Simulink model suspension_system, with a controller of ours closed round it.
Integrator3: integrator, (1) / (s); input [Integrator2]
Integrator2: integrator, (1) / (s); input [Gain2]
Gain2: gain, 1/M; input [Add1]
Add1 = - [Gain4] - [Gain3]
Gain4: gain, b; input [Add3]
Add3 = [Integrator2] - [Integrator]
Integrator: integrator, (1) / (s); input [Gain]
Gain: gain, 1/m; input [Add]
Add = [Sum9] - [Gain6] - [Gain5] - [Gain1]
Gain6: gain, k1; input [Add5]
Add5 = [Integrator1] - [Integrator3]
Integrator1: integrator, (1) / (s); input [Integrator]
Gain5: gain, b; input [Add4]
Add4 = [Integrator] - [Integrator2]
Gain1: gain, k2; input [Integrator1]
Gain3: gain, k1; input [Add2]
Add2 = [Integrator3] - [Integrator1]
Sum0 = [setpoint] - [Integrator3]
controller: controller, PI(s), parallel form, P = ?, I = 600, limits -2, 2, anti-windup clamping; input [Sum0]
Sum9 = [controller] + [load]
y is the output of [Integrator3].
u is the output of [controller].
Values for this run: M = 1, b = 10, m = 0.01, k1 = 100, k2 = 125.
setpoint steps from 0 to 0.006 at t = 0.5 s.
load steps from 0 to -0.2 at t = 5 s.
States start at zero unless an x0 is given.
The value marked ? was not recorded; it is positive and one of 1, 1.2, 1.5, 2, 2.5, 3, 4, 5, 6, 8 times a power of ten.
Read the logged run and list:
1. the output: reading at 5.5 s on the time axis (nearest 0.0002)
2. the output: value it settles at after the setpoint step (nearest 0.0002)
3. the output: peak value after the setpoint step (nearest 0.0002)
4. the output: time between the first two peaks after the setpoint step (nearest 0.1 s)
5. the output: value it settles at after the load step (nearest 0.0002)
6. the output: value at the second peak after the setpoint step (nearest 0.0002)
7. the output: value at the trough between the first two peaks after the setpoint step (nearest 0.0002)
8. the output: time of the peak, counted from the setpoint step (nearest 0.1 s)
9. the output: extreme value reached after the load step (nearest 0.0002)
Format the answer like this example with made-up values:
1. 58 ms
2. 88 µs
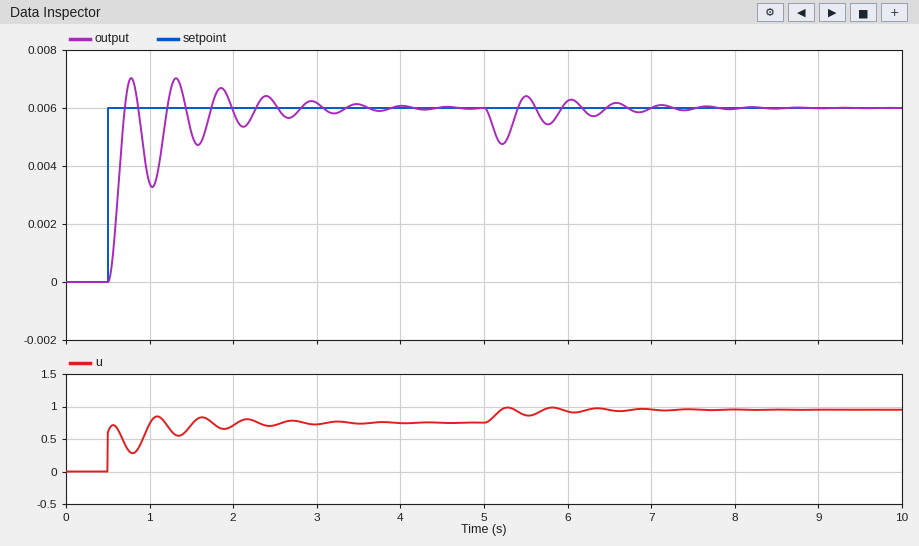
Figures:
1. 0.0064
2. 0.0060
3. 0.0070
4. 0.5 s
5. 0.0060
6. 0.0070
7. 0.0032
8. 0.3 s
9. 0.0048
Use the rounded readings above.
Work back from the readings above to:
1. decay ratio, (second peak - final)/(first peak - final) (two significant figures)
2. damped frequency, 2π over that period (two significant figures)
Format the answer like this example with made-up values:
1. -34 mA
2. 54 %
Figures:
1. 1.0
2. 13 rad/s
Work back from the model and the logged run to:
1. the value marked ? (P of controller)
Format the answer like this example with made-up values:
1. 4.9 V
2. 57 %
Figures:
1. 100
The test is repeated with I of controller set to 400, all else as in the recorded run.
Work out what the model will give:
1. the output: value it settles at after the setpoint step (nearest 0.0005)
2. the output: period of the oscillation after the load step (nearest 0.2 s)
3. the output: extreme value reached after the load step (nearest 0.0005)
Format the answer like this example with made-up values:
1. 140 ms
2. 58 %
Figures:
1. 0.0060
2. 0.6 s
3. 0.0045
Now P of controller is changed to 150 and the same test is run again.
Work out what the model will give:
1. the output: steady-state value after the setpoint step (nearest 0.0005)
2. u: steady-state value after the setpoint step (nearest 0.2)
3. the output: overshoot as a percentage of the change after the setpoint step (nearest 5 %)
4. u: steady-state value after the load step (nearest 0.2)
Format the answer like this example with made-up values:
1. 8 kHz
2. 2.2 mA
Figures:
1. 0.0060
2. 0.8
3. 20 %
4. 1.0
